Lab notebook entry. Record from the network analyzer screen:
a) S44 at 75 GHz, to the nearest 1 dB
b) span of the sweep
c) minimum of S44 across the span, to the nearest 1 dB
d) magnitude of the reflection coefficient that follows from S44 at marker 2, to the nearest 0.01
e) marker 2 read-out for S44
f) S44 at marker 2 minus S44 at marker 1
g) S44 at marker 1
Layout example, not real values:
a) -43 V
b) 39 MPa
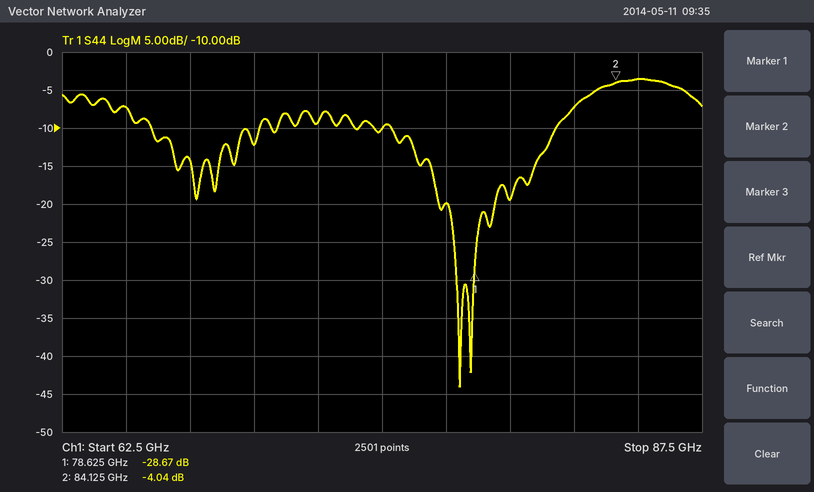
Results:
a) -10 dB
b) 25 GHz
c) -44 dB
d) 0.63
e) -4.04 dB
f) 24.63 dB
g) -28.67 dB
